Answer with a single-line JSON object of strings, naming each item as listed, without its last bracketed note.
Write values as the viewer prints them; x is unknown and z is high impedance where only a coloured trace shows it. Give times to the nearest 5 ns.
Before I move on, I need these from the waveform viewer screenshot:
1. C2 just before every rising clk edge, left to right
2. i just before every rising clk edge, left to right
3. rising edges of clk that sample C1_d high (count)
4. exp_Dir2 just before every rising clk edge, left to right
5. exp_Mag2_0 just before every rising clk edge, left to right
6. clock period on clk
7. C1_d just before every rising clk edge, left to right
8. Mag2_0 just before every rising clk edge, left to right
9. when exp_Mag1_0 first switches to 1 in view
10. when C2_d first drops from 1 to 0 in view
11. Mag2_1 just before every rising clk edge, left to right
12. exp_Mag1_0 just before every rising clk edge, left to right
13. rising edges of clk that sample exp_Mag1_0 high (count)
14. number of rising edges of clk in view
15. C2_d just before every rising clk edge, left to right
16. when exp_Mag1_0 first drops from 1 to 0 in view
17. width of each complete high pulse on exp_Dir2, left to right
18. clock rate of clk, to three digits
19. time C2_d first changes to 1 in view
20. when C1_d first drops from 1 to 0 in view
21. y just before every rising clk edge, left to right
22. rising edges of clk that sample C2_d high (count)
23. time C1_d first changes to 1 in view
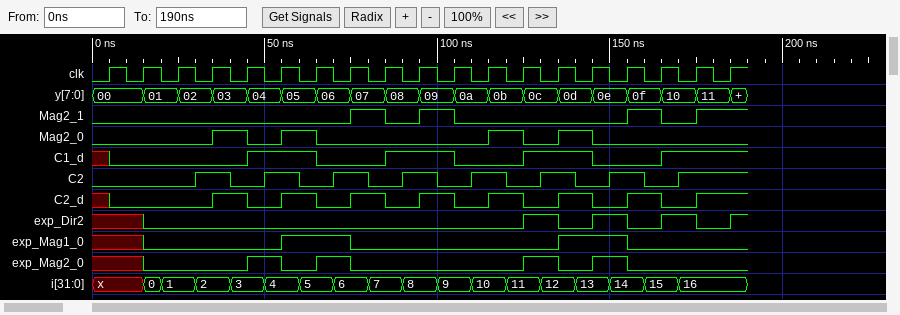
{"C2 just before every rising clk edge, left to right": "0 0 0 1 0 1 0 1 0 1 0 1 0 1 0 1 0 1 1", "i just before every rising clk edge, left to right": "x, x, 1, 2, 3, 4, 5, 6, 7, 8, 9, 10, 11, 12, 13, 14, 15, 16, 16", "rising edges of clk that sample C1_d high": "8", "exp_Dir2 just before every rising clk edge, left to right": "x x 0 0 0 0 0 0 0 0 0 0 0 1 0 1 0 1 0", "exp_Mag2_0 just before every rising clk edge, left to right": "x x 0 0 0 1 0 1 0 0 0 0 0 1 0 1 0 0 0", "clock period on clk": "10 ns", "C1_d just before every rising clk edge, left to right": "x 0 0 0 0 1 1 0 0 1 1 0 0 1 1 0 0 1 1", "Mag2_0 just before every rising clk edge, left to right": "0 0 0 0 1 0 1 0 0 0 0 0 1 0 1 0 0 0 0", "when exp_Mag1_0 first switches to 1 in view": "55 ns", "when C2_d first drops from 1 to 0 in view": "45 ns", "Mag2_1 just before every rising clk edge, left to right": "0 0 0 0 0 0 0 0 1 0 1 0 0 0 0 0 1 0 1", "exp_Mag1_0 just before every rising clk edge, left to right": "x x 0 0 0 0 1 1 0 0 0 0 0 0 1 1 0 0 0", "rising edges of clk that sample exp_Mag1_0 high": "4", "number of rising edges of clk in view": "19", "C2_d just before every rising clk edge, left to right": "x 0 0 0 1 0 1 0 1 0 1 0 1 0 1 0 1 0 1", "when exp_Mag1_0 first drops from 1 to 0 in view": "75 ns", "width of each complete high pulse on exp_Dir2, left to right": "10 ns, 10 ns, 10 ns", "clock rate of clk, to three digits": "100 MHz", "time C2_d first changes to 1 in view": "35 ns", "when C1_d first drops from 1 to 0 in view": "65 ns", "y just before every rising clk edge, left to right": "00, 00, 01, 02, 03, 04, 05, 06, 07, 08, 09, 0a, 0b, 0c, 0d, 0e, 0f, 10, 11", "rising edges of clk that sample C2_d high": "8", "time C1_d first changes to 1 in view": "45 ns"}
